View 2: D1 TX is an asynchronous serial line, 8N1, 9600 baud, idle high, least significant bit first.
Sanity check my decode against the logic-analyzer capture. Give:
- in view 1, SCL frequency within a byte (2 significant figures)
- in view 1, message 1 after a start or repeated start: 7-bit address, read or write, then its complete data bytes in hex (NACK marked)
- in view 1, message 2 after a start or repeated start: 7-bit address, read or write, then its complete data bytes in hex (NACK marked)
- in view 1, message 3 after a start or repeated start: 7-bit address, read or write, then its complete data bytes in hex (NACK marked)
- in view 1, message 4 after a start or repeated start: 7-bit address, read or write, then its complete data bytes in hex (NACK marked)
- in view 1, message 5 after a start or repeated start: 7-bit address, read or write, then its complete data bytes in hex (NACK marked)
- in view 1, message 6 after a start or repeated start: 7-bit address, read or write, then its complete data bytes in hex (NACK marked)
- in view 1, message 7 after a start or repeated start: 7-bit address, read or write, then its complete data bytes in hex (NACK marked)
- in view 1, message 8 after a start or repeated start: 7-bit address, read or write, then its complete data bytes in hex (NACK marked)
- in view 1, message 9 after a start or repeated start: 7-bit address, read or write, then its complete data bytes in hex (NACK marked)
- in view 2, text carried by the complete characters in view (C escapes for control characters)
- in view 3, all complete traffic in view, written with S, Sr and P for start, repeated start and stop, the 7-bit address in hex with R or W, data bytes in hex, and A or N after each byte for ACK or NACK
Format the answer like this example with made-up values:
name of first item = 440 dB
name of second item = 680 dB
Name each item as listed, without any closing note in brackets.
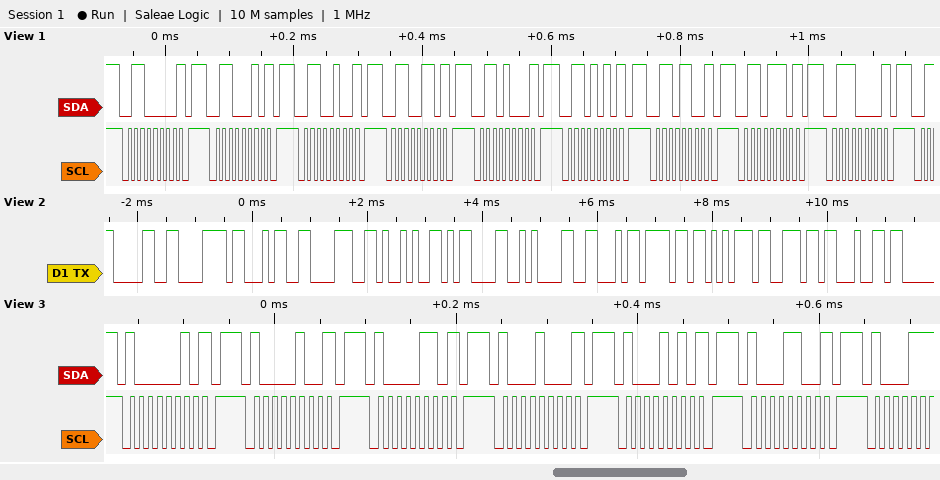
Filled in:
in view 1, SCL frequency within a byte = 100 kHz
in view 1, message 1 after a start or repeated start: 7-bit address, read or write, then its complete data bytes in hex = 0x30 write NACK
in view 1, message 2 after a start or repeated start: 7-bit address, read or write, then its complete data bytes in hex = 0x31 write NACK
in view 1, message 3 after a start or repeated start: 7-bit address, read or write, then its complete data bytes in hex = 0x32 write NACK
in view 1, message 4 after a start or repeated start: 7-bit address, read or write, then its complete data bytes in hex = 0x33 write NACK
in view 1, message 5 after a start or repeated start: 7-bit address, read or write, then its complete data bytes in hex = 0x34 write NACK
in view 1, message 6 after a start or repeated start: 7-bit address, read or write, then its complete data bytes in hex = 0x35 write NACK
in view 1, message 7 after a start or repeated start: 7-bit address, read or write, then its complete data bytes in hex = 0x36 write NACK
in view 1, message 8 after a start or repeated start: 7-bit address, read or write, then its complete data bytes in hex = 0x37 write NACK
in view 1, message 9 after a start or repeated start: 7-bit address, read or write, then its complete data bytes in hex = 0x38 write NACK
in view 2, text carried by the complete characters in view = "0x48)\r\nFound"
in view 3, all complete traffic in view, written with S, Sr and P for start, repeated start and stop, the 7-bit address in hex with R or W, data bytes in hex, and A or N after each byte for ACK or NACK = S 41W N P S 42W N P S 43W N P S 44W N P S 45W N P S 46W N P
